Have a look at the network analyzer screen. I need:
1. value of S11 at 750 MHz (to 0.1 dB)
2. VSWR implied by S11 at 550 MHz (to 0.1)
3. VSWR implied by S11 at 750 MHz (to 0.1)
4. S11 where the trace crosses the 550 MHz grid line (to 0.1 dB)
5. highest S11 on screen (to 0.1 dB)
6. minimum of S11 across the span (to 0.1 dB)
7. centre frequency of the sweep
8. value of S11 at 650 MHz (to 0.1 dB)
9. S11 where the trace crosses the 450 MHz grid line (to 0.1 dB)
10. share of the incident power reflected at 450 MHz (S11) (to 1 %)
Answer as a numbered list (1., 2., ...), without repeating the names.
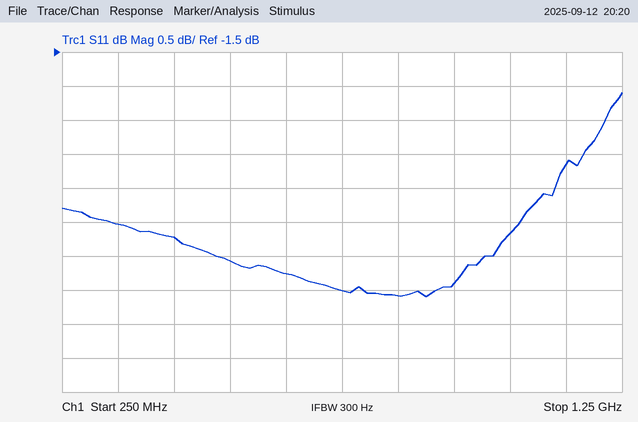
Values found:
1. -5.0 dB
2. 3.9
3. 3.6
4. -4.6 dB
5. -2.1 dB
6. -5.1 dB
7. 750 MHz
8. -4.8 dB
9. -4.2 dB
10. 38 %
